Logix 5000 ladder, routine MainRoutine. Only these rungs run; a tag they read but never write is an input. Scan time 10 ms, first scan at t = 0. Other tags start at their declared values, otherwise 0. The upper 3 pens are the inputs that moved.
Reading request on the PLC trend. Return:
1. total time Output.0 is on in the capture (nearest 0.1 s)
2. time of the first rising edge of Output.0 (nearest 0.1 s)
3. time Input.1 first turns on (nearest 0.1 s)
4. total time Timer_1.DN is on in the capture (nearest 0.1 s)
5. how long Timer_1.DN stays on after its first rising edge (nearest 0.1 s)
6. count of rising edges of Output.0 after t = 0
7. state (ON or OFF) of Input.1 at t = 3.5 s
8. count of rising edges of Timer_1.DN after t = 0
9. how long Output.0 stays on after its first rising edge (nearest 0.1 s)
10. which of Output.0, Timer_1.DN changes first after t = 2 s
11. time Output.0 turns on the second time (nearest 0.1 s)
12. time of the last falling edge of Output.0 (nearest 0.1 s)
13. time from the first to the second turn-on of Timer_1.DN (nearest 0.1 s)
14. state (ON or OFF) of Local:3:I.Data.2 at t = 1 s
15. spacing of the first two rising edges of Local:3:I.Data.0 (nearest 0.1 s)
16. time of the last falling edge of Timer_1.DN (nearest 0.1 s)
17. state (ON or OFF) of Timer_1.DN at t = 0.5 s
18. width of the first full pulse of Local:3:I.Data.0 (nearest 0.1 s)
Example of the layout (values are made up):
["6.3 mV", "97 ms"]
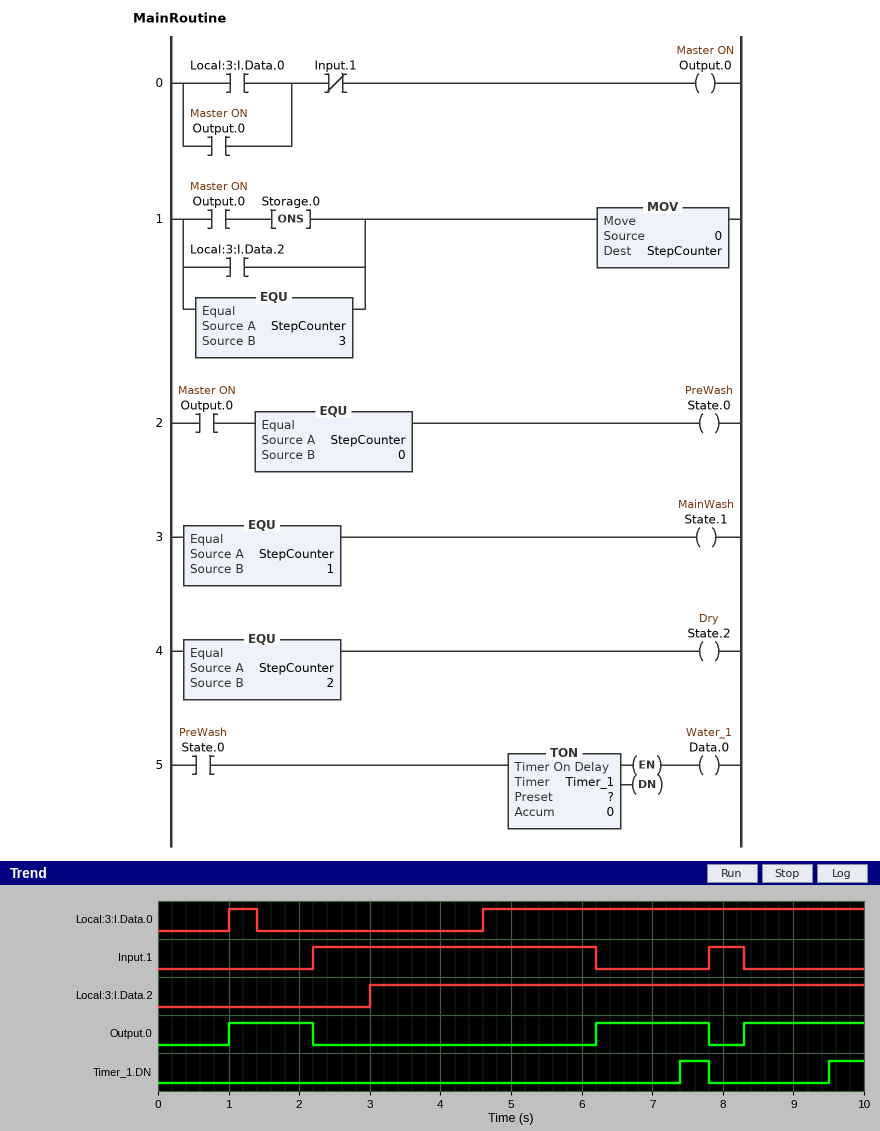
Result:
["4.5 s", "1.0 s", "2.2 s", "0.9 s", "0.4 s", "3", "ON", "2", "1.2 s", "Output.0", "6.2 s", "7.8 s", "2.1 s", "OFF", "3.6 s", "7.8 s", "OFF", "0.4 s"]
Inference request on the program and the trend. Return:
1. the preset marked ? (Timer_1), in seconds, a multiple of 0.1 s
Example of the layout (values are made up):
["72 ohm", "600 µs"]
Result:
["1.2 s"]
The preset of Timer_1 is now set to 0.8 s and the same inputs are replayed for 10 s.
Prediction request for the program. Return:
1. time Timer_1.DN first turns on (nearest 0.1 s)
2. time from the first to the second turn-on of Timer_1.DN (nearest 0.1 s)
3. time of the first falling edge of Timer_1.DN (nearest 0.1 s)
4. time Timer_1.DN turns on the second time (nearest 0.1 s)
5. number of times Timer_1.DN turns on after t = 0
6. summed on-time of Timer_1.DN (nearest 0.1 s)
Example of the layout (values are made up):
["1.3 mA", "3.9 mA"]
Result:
["1.8 s", "5.2 s", "2.2 s", "7.0 s", "3", "2.1 s"]
